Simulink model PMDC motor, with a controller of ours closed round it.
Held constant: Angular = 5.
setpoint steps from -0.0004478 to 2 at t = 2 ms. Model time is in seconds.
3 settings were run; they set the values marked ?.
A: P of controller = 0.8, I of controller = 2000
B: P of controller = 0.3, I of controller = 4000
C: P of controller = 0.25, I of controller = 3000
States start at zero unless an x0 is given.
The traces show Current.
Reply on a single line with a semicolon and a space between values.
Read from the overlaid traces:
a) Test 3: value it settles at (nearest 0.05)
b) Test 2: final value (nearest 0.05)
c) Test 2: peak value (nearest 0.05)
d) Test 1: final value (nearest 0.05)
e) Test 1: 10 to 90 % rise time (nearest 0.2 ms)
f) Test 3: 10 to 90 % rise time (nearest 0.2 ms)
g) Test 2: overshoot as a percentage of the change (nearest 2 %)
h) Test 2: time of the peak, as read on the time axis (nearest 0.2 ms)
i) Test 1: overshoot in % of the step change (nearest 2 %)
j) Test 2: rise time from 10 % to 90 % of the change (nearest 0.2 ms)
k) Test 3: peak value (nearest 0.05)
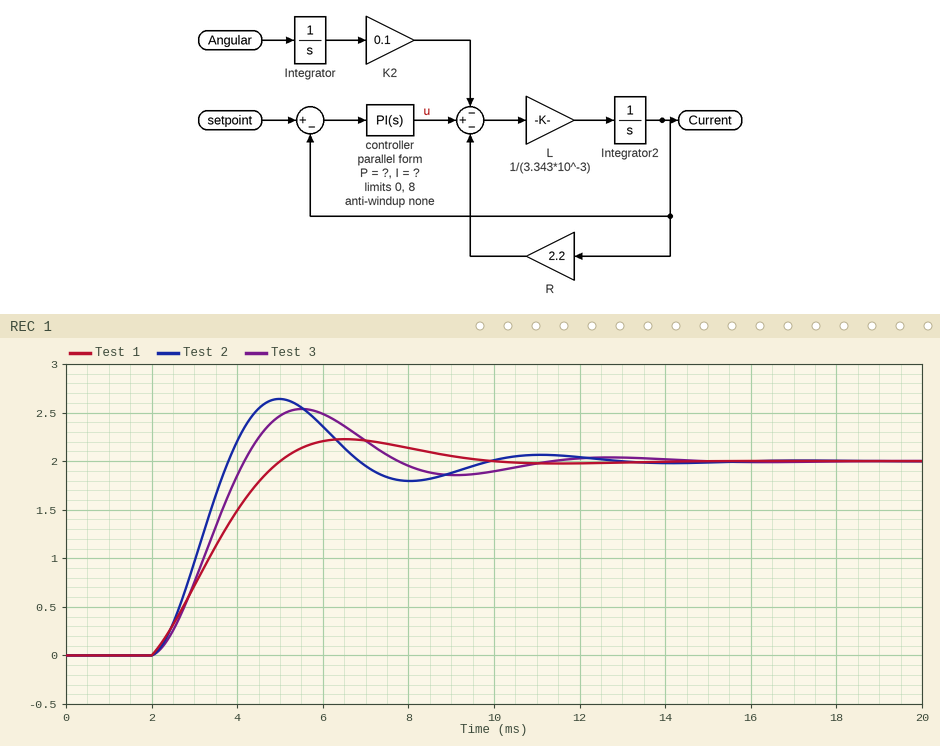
2.00; 2.00; 2.65; 2.00; 2.2 ms; 1.6 ms; 32 %; 5.0 ms; 12 %; 1.2 ms; 2.55
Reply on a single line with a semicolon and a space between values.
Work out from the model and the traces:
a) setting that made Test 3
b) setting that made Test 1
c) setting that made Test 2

C; A; B
